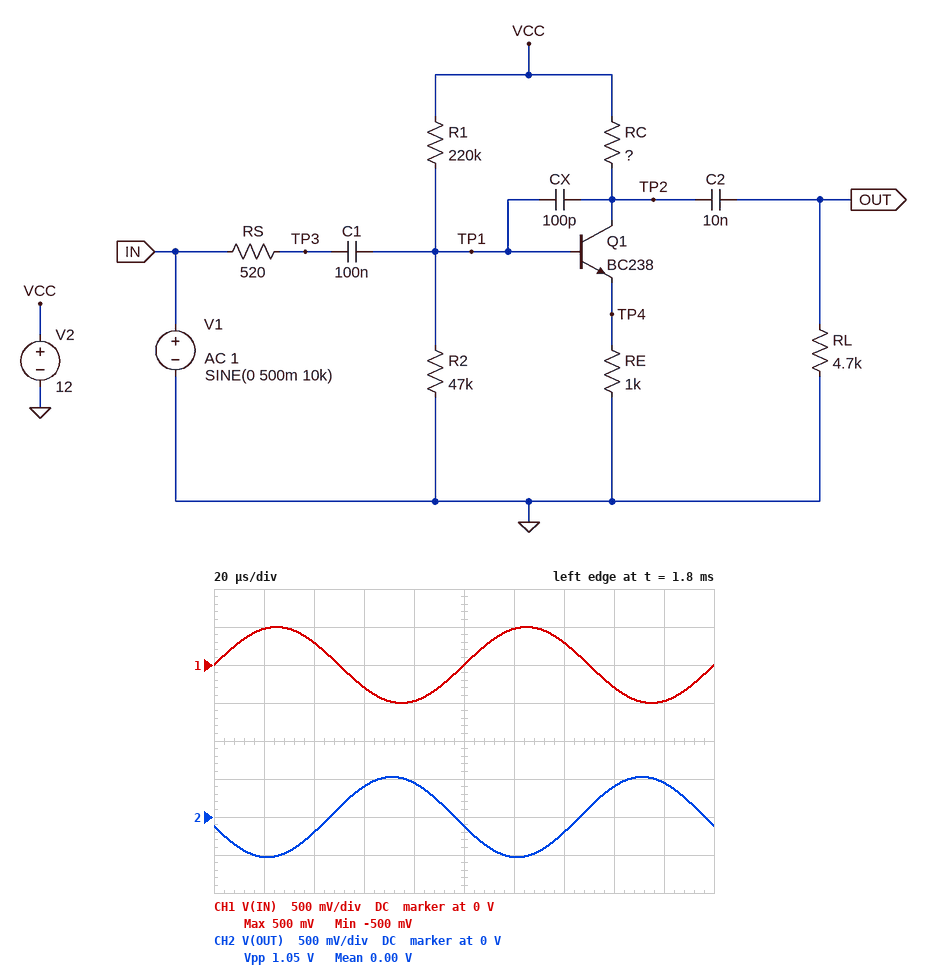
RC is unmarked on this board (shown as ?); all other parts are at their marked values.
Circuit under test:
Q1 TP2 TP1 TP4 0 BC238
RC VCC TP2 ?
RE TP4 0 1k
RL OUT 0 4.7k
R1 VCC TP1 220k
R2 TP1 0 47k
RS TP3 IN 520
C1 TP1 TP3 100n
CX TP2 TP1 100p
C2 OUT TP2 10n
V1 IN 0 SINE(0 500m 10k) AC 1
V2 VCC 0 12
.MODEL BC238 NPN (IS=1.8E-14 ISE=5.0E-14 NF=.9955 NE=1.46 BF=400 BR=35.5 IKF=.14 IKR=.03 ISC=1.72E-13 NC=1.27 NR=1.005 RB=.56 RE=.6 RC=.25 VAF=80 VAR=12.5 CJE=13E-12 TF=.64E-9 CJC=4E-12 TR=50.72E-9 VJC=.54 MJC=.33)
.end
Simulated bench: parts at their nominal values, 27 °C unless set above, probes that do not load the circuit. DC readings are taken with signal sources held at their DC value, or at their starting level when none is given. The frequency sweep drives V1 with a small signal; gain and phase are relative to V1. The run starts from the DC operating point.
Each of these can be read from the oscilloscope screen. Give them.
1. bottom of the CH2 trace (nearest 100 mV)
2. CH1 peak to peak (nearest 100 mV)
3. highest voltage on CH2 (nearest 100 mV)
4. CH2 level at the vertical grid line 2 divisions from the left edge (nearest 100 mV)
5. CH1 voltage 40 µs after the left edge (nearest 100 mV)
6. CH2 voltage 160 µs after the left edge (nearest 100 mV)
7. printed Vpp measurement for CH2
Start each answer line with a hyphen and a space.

- -500 mV
- 1.0 V
- 500 mV
- -200 mV
- 300 mV
- 400 mV
- 1.05 V
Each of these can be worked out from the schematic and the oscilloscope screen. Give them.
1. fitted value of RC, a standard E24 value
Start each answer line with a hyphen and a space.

- 1.5 kΩ
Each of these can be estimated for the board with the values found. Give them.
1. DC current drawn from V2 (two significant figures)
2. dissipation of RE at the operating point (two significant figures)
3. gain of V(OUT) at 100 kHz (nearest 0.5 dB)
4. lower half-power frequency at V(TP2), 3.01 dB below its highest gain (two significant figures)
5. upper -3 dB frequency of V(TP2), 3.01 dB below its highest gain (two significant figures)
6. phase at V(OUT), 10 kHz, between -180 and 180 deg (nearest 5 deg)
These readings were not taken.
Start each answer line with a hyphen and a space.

- 1.3 mA
- 1.7 mW
- 0.5 dB
- 44 Hz
- 340 kHz
- -165 deg
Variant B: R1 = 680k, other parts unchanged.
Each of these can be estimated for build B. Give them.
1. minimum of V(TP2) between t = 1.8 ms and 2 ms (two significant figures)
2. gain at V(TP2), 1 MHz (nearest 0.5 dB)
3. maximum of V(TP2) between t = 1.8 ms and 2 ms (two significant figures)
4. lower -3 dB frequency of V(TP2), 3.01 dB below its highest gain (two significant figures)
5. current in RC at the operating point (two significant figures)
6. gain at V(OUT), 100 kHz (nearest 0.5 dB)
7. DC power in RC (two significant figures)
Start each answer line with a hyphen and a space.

- 11 V
- -3.0 dB
- 12 V
- 40 Hz
- 160 µA
- -0.5 dB
- 38 µW
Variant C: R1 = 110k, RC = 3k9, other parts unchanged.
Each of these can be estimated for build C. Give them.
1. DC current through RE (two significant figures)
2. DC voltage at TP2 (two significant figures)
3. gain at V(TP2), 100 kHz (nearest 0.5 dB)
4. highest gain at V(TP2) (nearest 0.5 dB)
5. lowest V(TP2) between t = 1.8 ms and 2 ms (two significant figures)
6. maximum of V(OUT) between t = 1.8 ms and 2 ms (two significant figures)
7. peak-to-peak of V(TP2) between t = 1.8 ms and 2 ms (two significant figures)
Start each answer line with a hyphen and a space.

- 2.4 mA
- 2.5 V
- -1.0 dB
- 1.0 dB
- 2.6 V
- 960 mV
- 1.9 V
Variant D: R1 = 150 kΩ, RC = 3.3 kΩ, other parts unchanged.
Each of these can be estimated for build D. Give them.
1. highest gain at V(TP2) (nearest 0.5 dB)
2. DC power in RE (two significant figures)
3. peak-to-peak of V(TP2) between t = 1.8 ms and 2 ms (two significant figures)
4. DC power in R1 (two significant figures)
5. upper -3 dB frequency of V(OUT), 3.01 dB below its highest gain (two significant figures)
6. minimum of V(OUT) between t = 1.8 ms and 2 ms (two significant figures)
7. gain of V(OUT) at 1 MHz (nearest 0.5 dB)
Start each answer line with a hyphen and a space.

- 10.0 dB
- 3.9 mW
- 1.9 V
- 590 µW
- 510 kHz
- -910 mV
- -0.5 dB
